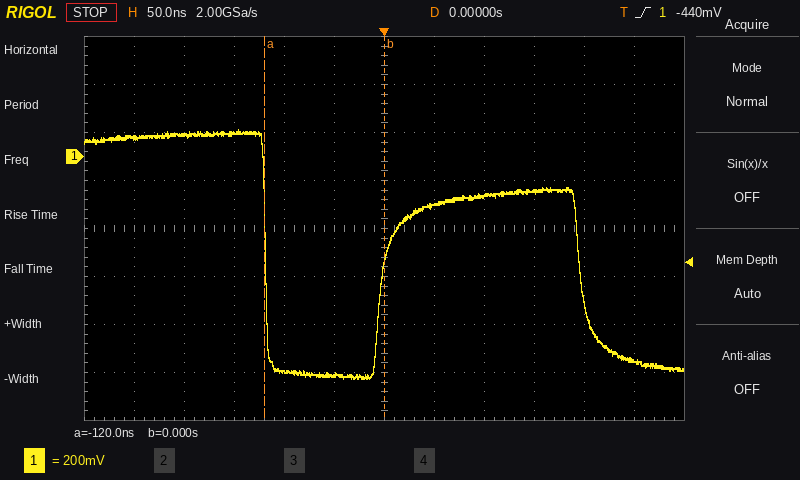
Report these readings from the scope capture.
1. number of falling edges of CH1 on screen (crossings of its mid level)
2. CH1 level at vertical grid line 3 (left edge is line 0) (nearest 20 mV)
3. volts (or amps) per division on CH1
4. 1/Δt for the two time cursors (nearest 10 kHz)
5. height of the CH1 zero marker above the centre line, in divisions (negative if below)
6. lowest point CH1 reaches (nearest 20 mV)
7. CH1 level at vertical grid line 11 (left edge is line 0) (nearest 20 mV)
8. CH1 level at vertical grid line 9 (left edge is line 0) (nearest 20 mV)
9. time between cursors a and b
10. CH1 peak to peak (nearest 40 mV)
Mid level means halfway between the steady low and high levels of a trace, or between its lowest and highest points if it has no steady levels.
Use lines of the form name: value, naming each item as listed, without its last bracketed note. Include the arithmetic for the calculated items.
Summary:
number of falling edges of CH1 on screen: 2
CH1 level at vertical grid line 3 (left edge is line 0): 100 mV
volts (or amps) per division on CH1: 200 mV
1/Δt for the two time cursors: 1 / 120 ns ≈ 8.33 MHz
height of the CH1 zero marker above the centre line, in divisions: +1.5 div
lowest point CH1 reaches: -920 mV
CH1 level at vertical grid line 11 (left edge is line 0): -860 mV
CH1 level at vertical grid line 9 (left edge is line 0): -140 mV
time between cursors a and b: 0 s − (-120 ns) = 120 ns
CH1 peak to peak: 1.04 V
